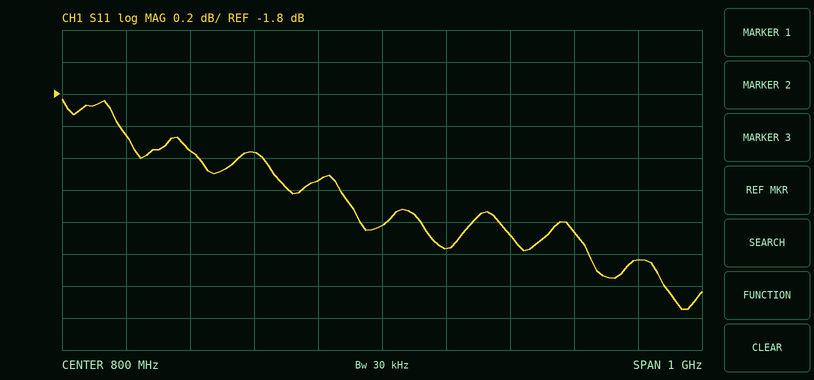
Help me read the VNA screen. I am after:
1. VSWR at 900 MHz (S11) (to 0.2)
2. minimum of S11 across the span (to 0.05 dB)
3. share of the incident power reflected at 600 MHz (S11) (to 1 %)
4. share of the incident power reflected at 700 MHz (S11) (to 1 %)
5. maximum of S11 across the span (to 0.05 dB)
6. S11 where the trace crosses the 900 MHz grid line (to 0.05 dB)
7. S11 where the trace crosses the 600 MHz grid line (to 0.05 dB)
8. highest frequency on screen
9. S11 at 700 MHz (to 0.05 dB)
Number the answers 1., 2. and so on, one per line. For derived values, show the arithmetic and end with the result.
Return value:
1. |Γ| = 10^(-2.75/20) = 0.7286; VSWR = (1 + 0.7286)/(1 − 0.7286) ≈ 6.4
2. -3.15 dB
3. 10^(-2.15/10) ≈ 61 %
4. 10^(-2.35/10) ≈ 58 %
5. -1.85 dB
6. -2.75 dB
7. -2.15 dB
8. 1.3 GHz
9. -2.35 dB
